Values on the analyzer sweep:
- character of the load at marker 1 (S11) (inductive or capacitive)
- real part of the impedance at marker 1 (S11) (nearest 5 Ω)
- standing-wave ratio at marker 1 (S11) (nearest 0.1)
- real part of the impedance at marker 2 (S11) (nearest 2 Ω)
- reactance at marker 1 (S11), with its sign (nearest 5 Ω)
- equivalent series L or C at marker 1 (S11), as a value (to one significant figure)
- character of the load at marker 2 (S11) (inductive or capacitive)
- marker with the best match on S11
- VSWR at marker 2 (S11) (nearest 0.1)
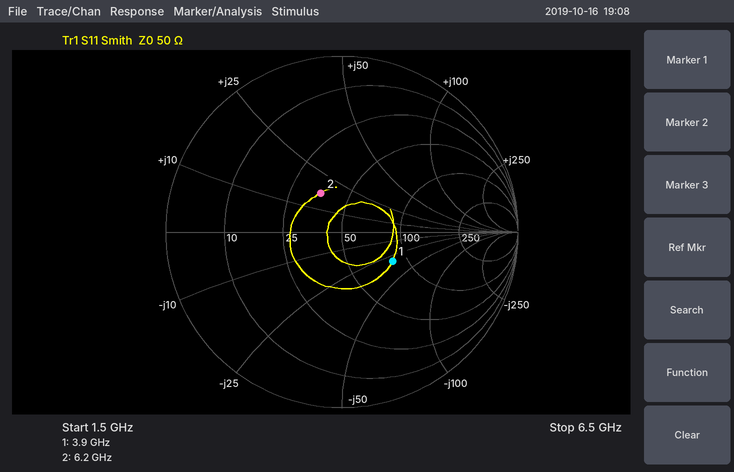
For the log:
capacitive
85 Ω
2.0
36 Ω
-30 Ω
1 pF
inductive
marker 2
1.7
